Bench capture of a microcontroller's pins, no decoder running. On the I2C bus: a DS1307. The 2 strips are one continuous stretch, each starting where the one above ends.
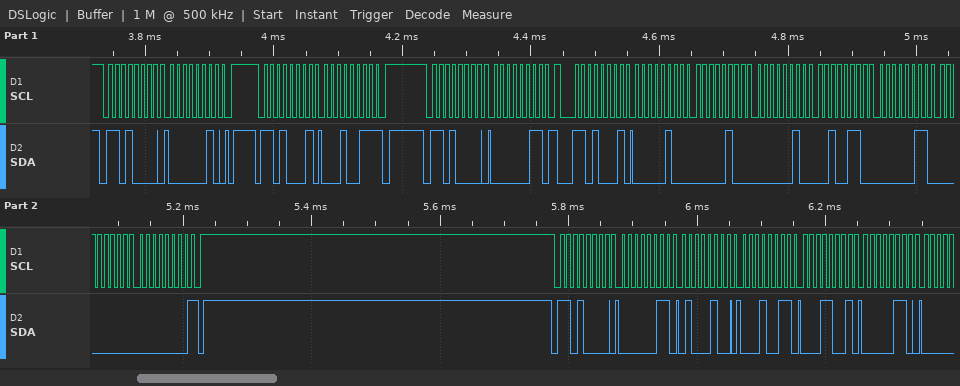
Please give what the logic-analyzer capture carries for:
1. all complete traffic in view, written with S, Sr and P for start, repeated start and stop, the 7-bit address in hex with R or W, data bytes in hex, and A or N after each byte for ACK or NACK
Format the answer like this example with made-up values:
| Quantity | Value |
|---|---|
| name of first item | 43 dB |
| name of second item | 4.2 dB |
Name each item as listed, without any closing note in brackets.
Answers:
| Quantity | Value |
|---|---|
| all complete traffic in view, written with S, Sr and P for start, repeated start and stop, the 7-bit address in hex with R or W, data bytes in hex, and A or N after each byte for ACK or NACK | S 68W A 02 A P S 68R A 13 N P S 68W A 03 A Sr 68R A 04 A 04 A 02 A 26 A 03 A 00 A 00 N P S 68W A 03 A 44 A 13 A 19 A 06 A |
